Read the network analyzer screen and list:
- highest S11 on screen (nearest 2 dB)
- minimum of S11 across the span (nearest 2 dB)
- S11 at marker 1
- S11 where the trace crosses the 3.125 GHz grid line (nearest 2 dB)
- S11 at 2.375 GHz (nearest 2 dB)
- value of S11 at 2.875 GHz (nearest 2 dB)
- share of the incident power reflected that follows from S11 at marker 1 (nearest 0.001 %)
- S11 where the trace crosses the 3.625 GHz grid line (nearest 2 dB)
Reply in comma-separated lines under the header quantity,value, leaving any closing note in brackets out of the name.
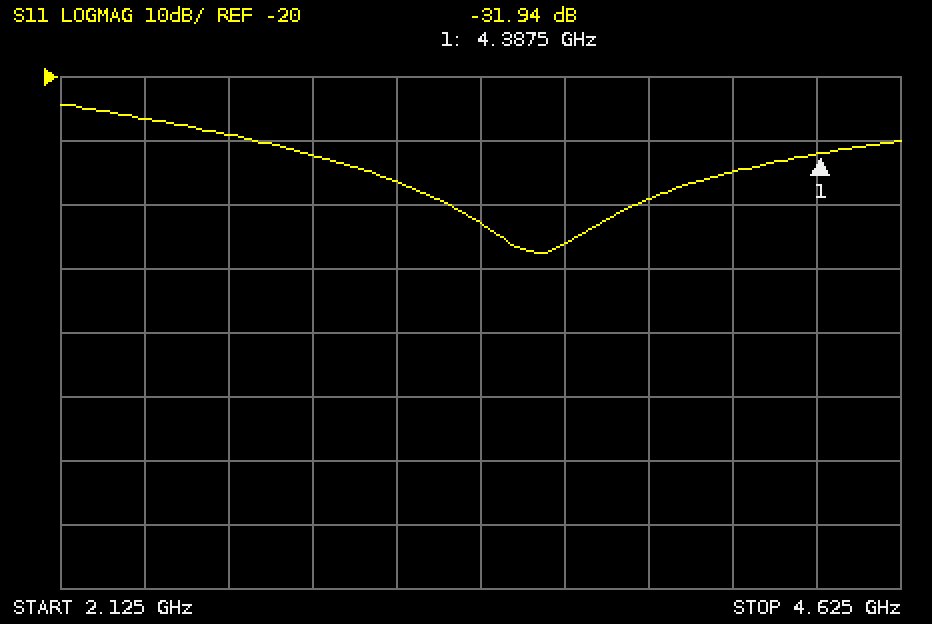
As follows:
quantity,value
highest S11 on screen,-24 dB
minimum of S11 across the span,-48 dB
S11 at marker 1,-31.94 dB
S11 where the trace crosses the 3.125 GHz grid line,-36 dB
S11 at 2.375 GHz,-26 dB
value of S11 at 2.875 GHz,-32 dB
share of the incident power reflected that follows from S11 at marker 1,0.064 %
S11 where the trace crosses the 3.625 GHz grid line,-46 dB
